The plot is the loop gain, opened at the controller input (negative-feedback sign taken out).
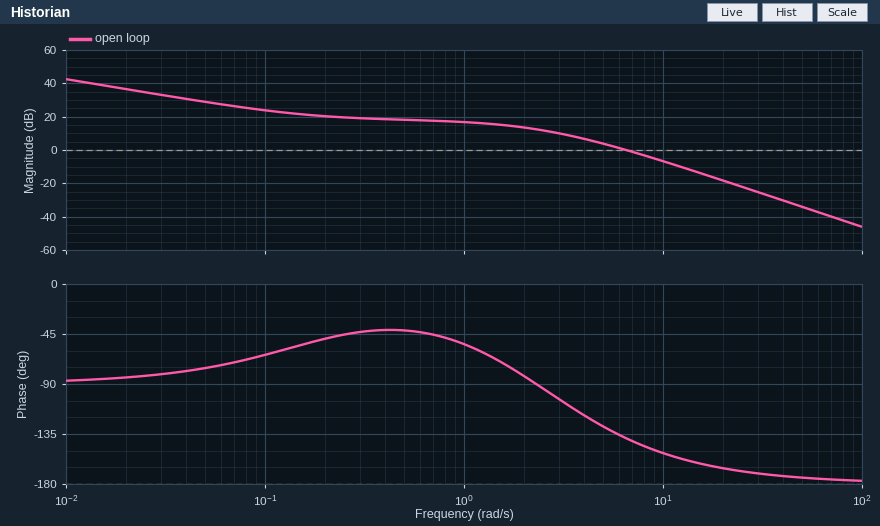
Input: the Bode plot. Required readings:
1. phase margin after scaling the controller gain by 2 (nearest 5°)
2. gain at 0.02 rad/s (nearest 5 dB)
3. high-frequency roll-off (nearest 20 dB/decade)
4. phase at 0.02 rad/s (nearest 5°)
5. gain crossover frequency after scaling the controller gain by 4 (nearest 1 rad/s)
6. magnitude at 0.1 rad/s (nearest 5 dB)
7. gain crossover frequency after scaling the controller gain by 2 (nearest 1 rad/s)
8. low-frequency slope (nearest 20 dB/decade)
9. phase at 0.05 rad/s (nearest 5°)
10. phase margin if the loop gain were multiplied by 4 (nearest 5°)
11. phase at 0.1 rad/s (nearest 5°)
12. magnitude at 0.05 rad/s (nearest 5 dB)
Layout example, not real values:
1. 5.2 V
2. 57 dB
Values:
1. 30°
2. 35 dB
3. -40 dB/decade
4. -85°
5. 14 rad/s
6. 25 dB
7. 10 rad/s
8. -20 dB/decade
9. -75°
10. 20°
11. -65°
12. 30 dB
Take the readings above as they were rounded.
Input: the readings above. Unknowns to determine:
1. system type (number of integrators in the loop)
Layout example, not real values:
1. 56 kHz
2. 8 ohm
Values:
1. 1
